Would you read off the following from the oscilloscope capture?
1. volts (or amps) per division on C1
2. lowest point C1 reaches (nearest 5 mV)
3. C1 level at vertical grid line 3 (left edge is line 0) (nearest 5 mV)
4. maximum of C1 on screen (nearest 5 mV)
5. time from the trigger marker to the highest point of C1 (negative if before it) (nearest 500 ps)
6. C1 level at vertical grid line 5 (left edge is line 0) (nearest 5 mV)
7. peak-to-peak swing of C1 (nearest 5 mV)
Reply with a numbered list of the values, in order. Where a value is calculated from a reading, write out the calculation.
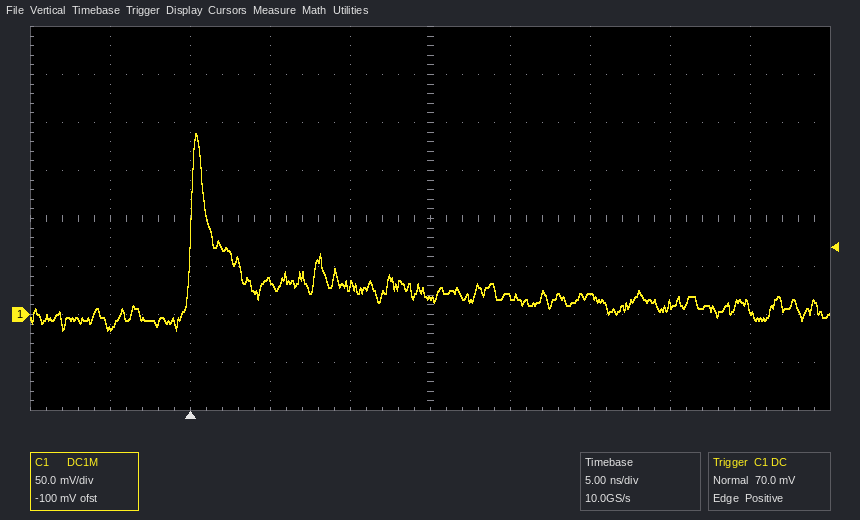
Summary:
1. 50 mV
2. -15 mV
3. 35 mV
4. 190 mV
5. +500 ps
6. 15 mV
7. 190 mV − (-15 mV) = 205 mV
